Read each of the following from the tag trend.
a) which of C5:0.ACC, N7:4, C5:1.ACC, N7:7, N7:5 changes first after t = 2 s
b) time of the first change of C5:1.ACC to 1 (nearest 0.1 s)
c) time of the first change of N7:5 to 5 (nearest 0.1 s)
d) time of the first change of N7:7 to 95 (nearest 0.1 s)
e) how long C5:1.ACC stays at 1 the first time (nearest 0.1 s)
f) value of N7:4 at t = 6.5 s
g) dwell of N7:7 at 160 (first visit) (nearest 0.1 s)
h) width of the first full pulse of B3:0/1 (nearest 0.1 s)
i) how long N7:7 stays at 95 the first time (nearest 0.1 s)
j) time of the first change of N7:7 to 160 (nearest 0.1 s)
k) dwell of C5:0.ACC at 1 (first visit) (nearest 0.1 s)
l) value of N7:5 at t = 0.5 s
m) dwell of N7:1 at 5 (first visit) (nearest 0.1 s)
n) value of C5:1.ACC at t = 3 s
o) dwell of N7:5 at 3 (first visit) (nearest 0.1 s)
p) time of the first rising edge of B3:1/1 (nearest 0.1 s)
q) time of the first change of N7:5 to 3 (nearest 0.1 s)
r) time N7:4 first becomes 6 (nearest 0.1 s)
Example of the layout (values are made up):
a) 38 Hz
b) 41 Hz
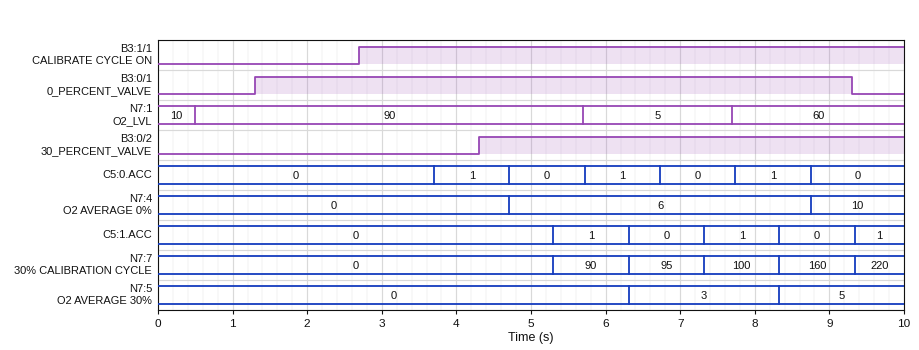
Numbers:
a) C5:0.ACC
b) 5.3 s
c) 8.3 s
d) 6.3 s
e) 1.0 s
f) 6
g) 1.0 s
h) 8.0 s
i) 1.0 s
j) 8.3 s
k) 1.0 s
l) 0
m) 2.0 s
n) 0
o) 2.0 s
p) 2.7 s
q) 6.3 s
r) 4.7 s
